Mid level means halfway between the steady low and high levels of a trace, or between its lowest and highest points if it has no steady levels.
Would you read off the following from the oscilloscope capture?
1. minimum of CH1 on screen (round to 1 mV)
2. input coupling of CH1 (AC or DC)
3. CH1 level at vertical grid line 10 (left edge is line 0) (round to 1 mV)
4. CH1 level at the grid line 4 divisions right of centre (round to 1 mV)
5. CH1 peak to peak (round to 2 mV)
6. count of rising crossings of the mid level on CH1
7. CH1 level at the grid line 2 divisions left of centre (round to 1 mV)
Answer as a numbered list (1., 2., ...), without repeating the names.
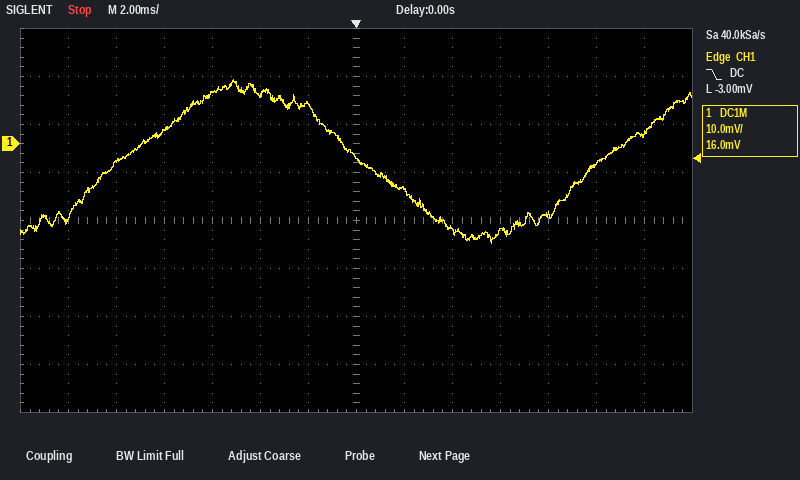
1. -21 mV
2. DC
3. -18 mV
4. -15 mV
5. 34 mV
6. 2
7. 10 mV
